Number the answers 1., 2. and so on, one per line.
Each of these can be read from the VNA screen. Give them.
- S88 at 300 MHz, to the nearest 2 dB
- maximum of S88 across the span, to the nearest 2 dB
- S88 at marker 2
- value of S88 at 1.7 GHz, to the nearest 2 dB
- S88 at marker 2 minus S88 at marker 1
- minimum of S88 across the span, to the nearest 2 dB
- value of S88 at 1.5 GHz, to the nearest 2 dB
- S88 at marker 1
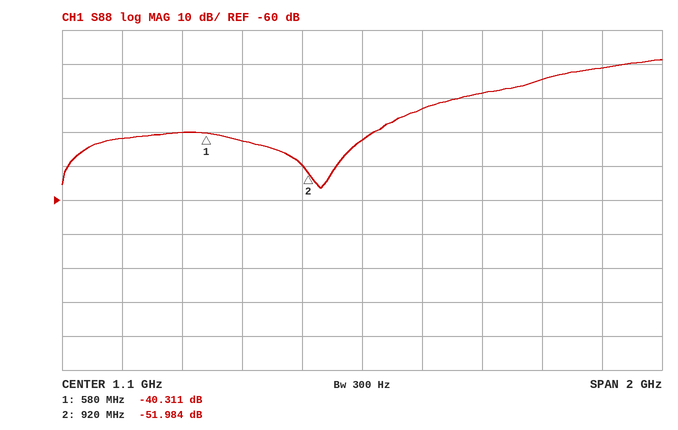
1. -42 dB
2. -18 dB
3. -51.984 dB
4. -24 dB
5. -11.673 dB
6. -56 dB
7. -28 dB
8. -40.311 dB
